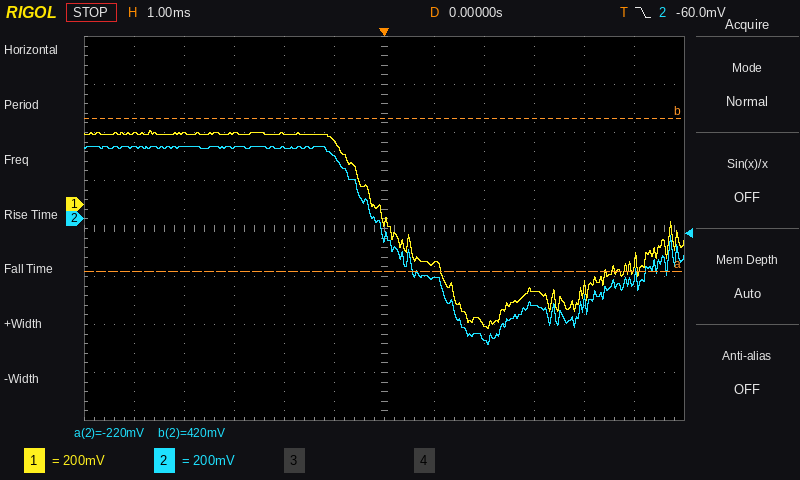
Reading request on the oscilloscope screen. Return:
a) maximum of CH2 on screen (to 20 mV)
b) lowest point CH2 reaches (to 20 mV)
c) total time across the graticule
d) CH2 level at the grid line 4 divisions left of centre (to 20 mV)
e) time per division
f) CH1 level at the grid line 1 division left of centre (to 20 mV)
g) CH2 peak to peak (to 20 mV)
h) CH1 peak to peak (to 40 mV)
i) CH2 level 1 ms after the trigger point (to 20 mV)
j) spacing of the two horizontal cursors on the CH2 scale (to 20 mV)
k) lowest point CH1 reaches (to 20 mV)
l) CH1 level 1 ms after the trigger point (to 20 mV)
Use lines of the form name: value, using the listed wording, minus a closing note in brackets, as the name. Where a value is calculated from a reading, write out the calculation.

maximum of CH2 on screen: 300 mV
lowest point CH2 reaches: -520 mV
total time across the graticule: 12 ms
CH2 level at the grid line 4 divisions left of centre: 300 mV
time per division: 1 ms
CH1 level at the grid line 1 division left of centre: 260 mV
CH2 peak to peak: 300 mV − (-520 mV) = 820 mV
CH1 peak to peak: 840 mV
CH2 level 1 ms after the trigger point: -240 mV
spacing of the two horizontal cursors on the CH2 scale: 640 mV
lowest point CH1 reaches: -520 mV
CH1 level 1 ms after the trigger point: -240 mV
